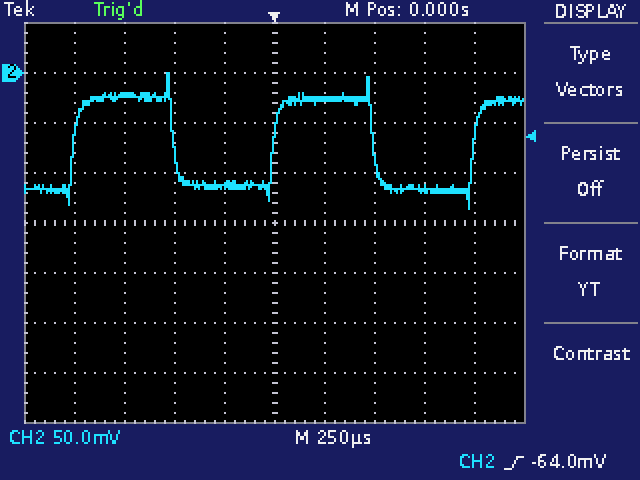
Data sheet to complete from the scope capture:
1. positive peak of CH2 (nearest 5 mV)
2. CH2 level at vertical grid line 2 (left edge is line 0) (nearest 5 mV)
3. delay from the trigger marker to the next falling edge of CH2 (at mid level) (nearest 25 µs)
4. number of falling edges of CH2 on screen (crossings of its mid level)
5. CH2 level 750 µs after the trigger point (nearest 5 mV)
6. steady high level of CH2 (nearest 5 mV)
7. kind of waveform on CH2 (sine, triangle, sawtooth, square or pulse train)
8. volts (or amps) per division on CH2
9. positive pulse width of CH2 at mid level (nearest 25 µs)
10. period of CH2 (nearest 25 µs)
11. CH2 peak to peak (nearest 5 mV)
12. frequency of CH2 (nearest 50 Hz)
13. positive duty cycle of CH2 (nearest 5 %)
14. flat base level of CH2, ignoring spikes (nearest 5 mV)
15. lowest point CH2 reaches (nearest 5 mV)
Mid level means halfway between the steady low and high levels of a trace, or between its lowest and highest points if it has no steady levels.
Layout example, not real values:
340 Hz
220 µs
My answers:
0 mV
-20 mV
500 µs
2
-115 mV
-25 mV
square
50 mV
500 µs
1.000 ms
135 mV
1.00 kHz
50 %
-115 mV
-135 mV
